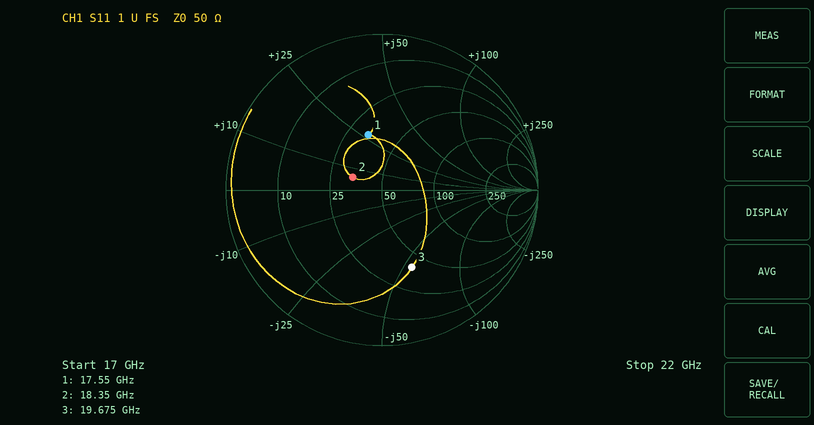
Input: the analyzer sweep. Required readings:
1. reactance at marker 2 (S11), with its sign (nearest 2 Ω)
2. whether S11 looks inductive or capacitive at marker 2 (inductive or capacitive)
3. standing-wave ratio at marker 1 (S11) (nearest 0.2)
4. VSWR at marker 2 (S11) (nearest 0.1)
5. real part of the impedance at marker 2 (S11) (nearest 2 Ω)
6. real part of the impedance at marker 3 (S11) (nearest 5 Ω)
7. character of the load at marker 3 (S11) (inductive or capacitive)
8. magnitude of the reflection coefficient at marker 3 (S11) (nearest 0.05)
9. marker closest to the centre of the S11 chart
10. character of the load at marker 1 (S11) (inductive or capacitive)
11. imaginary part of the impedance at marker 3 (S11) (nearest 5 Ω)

+6 Ω
inductive
2.2
1.5
34 Ω
40 Ω
capacitive
0.55
marker 2
inductive
-55 Ω
